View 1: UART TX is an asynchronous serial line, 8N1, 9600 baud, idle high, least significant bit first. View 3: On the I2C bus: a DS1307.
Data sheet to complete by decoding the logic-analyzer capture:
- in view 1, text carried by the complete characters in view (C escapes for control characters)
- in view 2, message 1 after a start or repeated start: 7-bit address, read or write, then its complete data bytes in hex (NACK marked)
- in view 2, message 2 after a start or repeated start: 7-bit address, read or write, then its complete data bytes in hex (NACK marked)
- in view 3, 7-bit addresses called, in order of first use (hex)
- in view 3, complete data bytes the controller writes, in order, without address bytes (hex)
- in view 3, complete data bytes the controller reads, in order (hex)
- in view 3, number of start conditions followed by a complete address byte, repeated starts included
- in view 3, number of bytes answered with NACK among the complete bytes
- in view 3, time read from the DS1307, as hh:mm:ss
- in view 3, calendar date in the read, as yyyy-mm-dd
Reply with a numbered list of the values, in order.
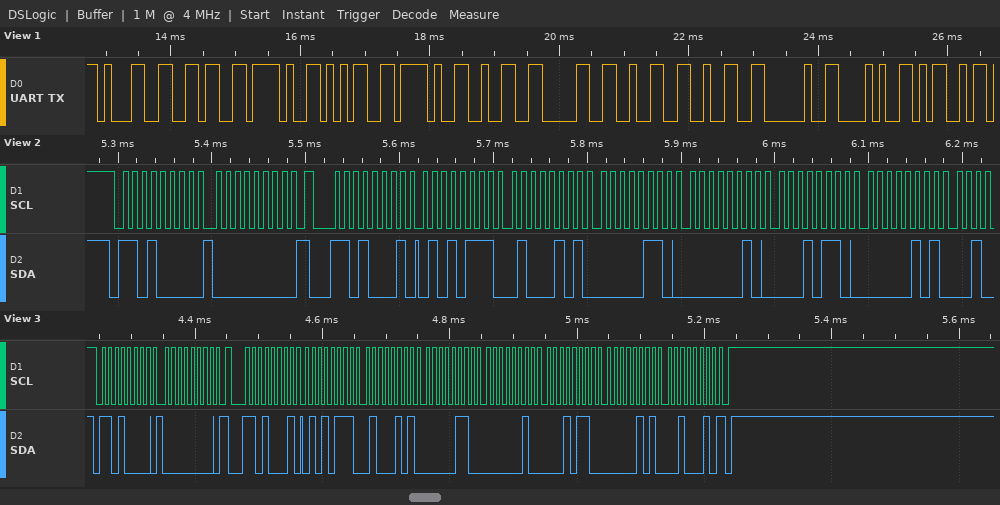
1. "16/5/2022 (M"
2. 0x68 write: 00
3. 0x68 read: 57 45 06 02 16 05
4. 0x68
5. 00
6. 57 45 06 02 16 05 22
7. 2
8. 1
9. 06:45:57
10. 2022-05-16
